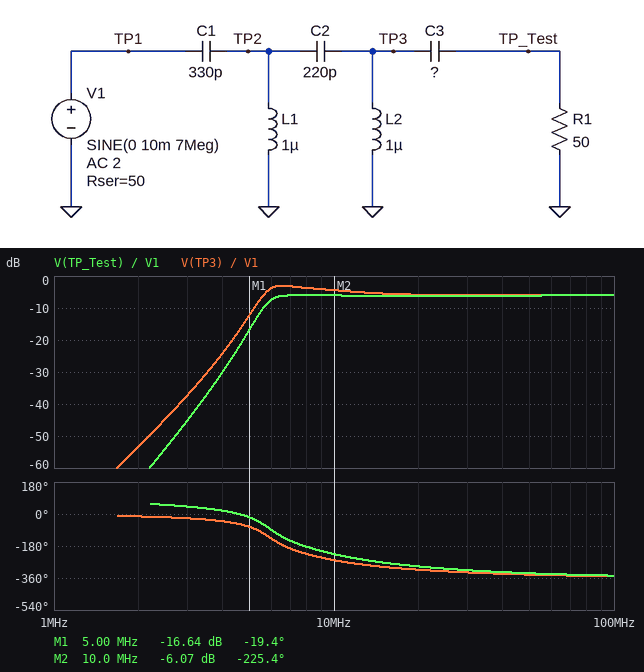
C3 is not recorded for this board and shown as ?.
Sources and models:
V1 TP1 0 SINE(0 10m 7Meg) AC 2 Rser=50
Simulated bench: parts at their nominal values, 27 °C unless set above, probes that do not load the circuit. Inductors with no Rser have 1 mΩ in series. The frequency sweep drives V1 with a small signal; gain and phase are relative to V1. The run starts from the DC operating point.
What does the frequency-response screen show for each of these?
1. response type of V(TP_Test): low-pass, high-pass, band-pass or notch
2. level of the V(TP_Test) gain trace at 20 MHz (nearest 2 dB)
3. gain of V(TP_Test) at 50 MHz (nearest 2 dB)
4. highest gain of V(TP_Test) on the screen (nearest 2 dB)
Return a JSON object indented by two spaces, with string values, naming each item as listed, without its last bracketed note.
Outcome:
{
  "response type of V(TP_Test): low-pass, high-pass, band-pass or notch": "high-pass",
  "level of the V(TP_Test) gain trace at 20 MHz": "-6 dB",
  "gain of V(TP_Test) at 50 MHz": "-6 dB",
  "highest gain of V(TP_Test) on the screen": "-6 dB"
}
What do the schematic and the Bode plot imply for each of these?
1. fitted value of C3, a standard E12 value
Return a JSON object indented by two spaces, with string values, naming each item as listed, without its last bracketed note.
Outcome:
{
  "fitted value of C3, a standard E12 value": "470 pF"
}
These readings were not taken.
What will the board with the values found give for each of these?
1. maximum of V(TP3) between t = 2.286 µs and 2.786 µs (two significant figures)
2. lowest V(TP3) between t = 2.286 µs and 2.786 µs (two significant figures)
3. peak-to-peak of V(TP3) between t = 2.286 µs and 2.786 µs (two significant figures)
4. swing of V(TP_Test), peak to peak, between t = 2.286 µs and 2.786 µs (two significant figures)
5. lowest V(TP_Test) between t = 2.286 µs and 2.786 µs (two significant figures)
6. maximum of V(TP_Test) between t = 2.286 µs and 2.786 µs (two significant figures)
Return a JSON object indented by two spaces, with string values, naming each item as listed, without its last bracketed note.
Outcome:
{
  "maximum of V(TP3) between t = 2.286 µs and 2.786 µs": "6.9 mV",
  "lowest V(TP3) between t = 2.286 µs and 2.786 µs": "-6.9 mV",
  "peak-to-peak of V(TP3) between t = 2.286 µs and 2.786 µs": "14 mV",
  "swing of V(TP_Test), peak to peak, between t = 2.286 µs and 2.786 µs": "9.9 mV",
  "lowest V(TP_Test) between t = 2.286 µs and 2.786 µs": "-5.0 mV",
  "maximum of V(TP_Test) between t = 2.286 µs and 2.786 µs": "5.0 mV"
}
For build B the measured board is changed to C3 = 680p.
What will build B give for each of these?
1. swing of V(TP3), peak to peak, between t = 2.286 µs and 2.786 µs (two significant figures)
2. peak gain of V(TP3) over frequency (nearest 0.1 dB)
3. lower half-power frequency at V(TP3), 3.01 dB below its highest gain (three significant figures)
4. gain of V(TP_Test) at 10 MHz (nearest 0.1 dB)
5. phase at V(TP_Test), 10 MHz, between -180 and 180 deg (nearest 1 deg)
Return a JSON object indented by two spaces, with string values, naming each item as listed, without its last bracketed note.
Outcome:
{
  "swing of V(TP3), peak to peak, between t = 2.286 µs and 2.786 µs": "12 mV",
  "peak gain of V(TP3) over frequency": "-4.5 dB",
  "lower half-power frequency at V(TP3), 3.01 dB below its highest gain": "5.68 MHz",
  "gain of V(TP_Test) at 10 MHz": "-6.2 dB",
  "phase at V(TP_Test), 10 MHz, between -180 and 180 deg": "128 deg"
}
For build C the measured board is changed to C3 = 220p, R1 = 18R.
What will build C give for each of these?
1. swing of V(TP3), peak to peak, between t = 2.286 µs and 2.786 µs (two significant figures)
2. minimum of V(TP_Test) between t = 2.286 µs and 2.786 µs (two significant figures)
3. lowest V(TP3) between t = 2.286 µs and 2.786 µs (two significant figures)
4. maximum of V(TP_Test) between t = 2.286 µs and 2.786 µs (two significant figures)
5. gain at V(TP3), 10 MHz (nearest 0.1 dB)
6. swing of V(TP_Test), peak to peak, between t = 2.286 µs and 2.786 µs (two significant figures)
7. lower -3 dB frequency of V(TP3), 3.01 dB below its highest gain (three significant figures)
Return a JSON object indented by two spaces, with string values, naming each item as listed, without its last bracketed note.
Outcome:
{
  "swing of V(TP3), peak to peak, between t = 2.286 µs and 2.786 µs": "23 mV",
  "minimum of V(TP_Test) between t = 2.286 µs and 2.786 µs": "-2.0 mV",
  "lowest V(TP3) between t = 2.286 µs and 2.786 µs": "-12 mV",
  "maximum of V(TP_Test) between t = 2.286 µs and 2.786 µs": "2.0 mV",
  "gain at V(TP3), 10 MHz": "0.1 dB",
  "swing of V(TP_Test), peak to peak, between t = 2.286 µs and 2.786 µs": "4.0 mV",
  "lower -3 dB frequency of V(TP3), 3.01 dB below its highest gain": "5.89 MHz"
}
